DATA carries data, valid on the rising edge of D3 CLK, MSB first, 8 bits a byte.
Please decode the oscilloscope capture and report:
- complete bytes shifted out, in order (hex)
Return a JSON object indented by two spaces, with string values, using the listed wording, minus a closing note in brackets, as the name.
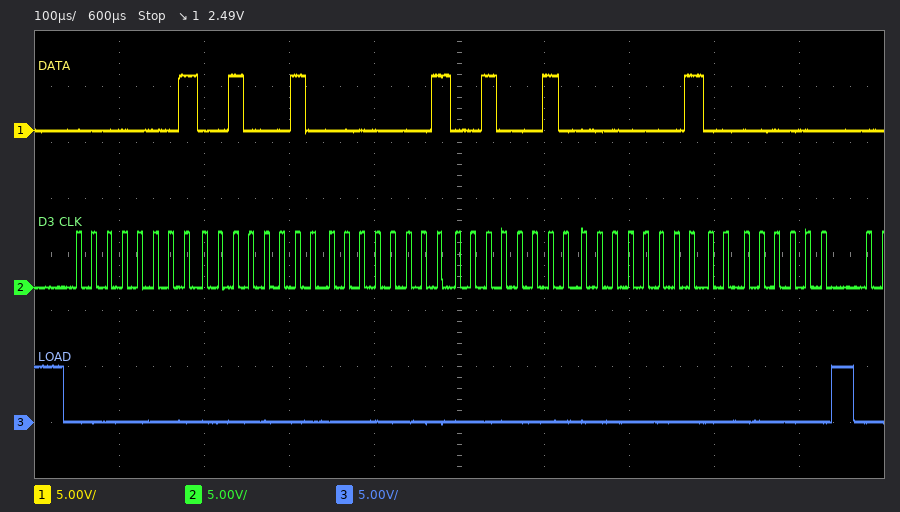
{
  "complete bytes shifted out, in order": "01 22 01 22 01 00"
}
